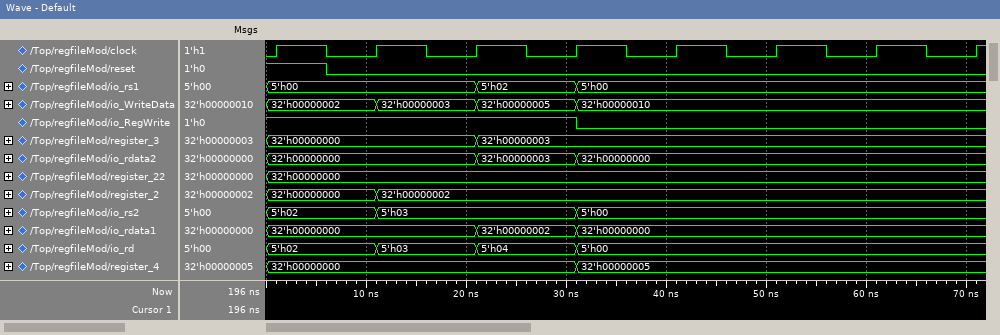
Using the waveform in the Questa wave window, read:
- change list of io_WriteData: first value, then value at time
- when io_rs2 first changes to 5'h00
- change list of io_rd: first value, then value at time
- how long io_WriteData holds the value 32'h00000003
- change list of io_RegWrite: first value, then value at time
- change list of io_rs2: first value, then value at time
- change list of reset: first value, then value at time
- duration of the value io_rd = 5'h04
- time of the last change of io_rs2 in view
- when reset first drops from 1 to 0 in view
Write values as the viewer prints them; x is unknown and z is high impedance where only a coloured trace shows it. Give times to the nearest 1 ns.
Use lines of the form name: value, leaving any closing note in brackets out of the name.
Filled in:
change list of io_WriteData: first value, then value at time: 32'h00000002, 32'h00000003 at 11 ns, 32'h00000005 at 21 ns, 32'h00000010 at 31 ns
when io_rs2 first changes to 5'h00: 31 ns
change list of io_rd: first value, then value at time: 5'h02, 5'h03 at 11 ns, 5'h04 at 21 ns, 5'h00 at 31 ns
how long io_WriteData holds the value 32'h00000003: 10 ns
change list of io_RegWrite: first value, then value at time: 1, 0 at 31 ns
change list of io_rs2: first value, then value at time: 5'h02, 5'h03 at 11 ns, 5'h00 at 31 ns
change list of reset: first value, then value at time: 1, 0 at 6 ns
duration of the value io_rd = 5'h04: 10 ns
time of the last change of io_rs2 in view: 31 ns
when reset first drops from 1 to 0 in view: 6 ns
